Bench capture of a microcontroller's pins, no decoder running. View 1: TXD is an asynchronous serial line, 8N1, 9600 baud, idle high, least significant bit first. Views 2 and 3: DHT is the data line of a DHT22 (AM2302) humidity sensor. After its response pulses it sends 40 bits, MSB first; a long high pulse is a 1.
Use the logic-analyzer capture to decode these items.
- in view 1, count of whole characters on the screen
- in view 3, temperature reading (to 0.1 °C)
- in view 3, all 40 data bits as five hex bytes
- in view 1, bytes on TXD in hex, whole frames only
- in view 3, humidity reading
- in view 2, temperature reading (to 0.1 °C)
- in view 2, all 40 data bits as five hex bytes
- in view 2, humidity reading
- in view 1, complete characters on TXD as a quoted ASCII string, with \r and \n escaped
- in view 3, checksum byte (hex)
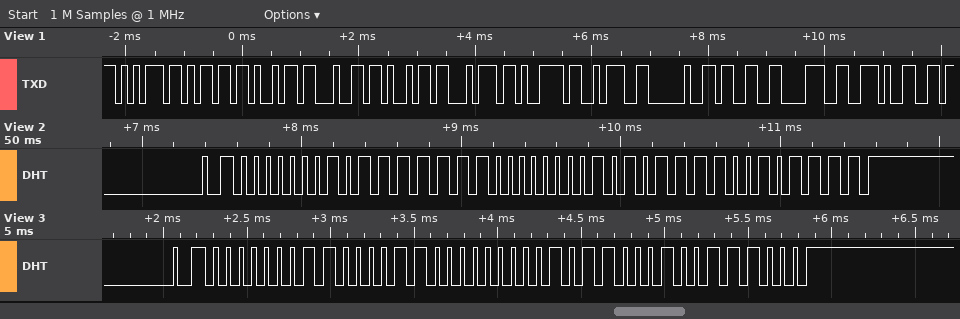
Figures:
12
17.7 °C
01 86 00 B1 38
75 6D 69 64 69 74 79 3A 20 33 38 2E
39.0 %
17.5 °C
01 7F 00 AF 2F
38.3 %
"umidity: 38."
0x38
